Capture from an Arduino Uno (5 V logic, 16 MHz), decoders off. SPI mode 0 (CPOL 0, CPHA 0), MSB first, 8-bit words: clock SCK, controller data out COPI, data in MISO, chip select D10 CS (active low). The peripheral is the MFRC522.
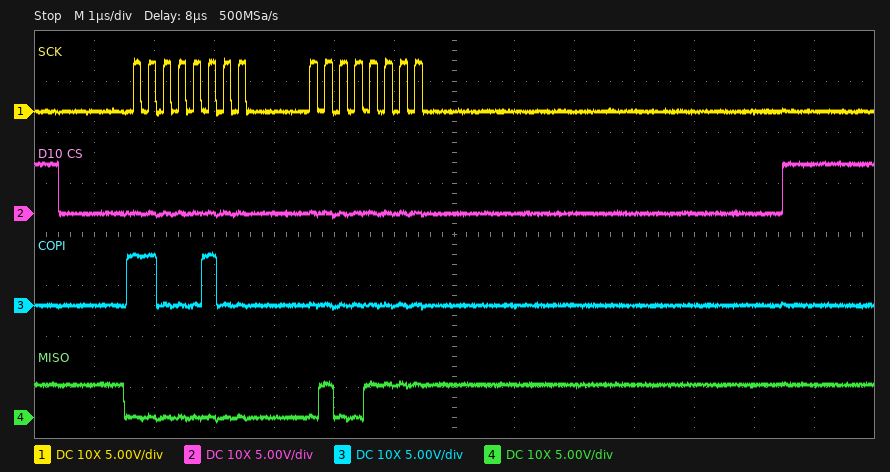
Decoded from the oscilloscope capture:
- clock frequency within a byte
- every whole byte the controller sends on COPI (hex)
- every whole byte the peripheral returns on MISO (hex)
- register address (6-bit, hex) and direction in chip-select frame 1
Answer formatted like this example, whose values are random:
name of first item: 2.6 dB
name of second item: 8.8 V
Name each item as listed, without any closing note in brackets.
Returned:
clock frequency within a byte: 4 MHz
every whole byte the controller sends on COPI: C4 00
every whole byte the peripheral returns on MISO: 00 4F
register address (6-bit, hex) and direction in chip-select frame 1: 0x22 read
